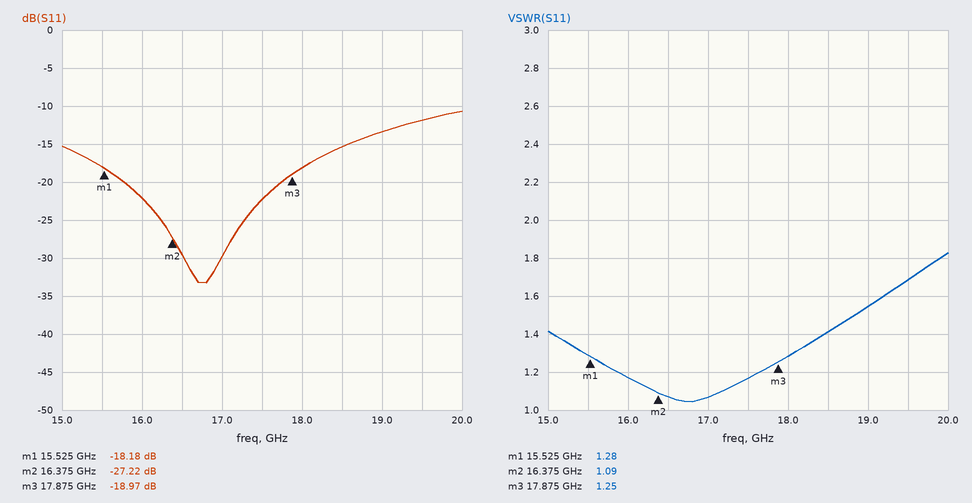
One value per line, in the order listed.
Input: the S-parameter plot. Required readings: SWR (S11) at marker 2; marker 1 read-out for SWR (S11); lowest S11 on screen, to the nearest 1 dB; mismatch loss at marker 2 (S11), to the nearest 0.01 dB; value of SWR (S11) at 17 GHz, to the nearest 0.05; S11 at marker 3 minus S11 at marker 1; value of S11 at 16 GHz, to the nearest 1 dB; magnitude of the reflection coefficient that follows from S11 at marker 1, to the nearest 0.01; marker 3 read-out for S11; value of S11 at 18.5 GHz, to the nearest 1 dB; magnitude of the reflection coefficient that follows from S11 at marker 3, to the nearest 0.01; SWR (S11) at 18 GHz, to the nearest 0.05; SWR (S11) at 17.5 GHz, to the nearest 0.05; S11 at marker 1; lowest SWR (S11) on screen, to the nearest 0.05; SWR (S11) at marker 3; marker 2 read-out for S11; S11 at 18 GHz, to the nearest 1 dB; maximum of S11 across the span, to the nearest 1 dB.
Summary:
1.09
1.28
-33 dB
0.01 dB
1.05
-0.79 dB
-22 dB
0.12
-18.97 dB
-15 dB
0.11
1.30
1.15
-18.18 dB
1.05
1.25
-27.22 dB
-18 dB
-11 dB
